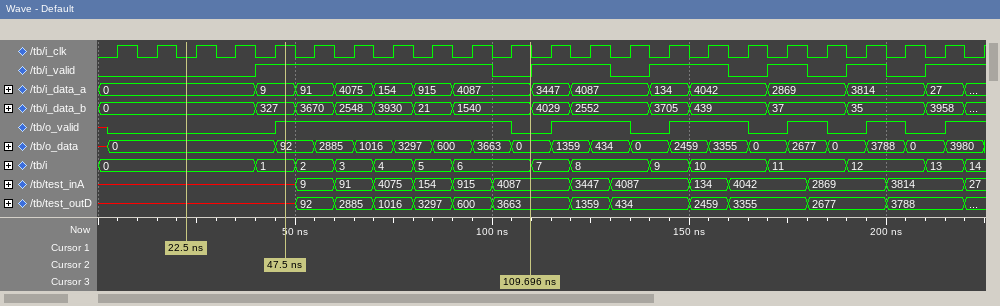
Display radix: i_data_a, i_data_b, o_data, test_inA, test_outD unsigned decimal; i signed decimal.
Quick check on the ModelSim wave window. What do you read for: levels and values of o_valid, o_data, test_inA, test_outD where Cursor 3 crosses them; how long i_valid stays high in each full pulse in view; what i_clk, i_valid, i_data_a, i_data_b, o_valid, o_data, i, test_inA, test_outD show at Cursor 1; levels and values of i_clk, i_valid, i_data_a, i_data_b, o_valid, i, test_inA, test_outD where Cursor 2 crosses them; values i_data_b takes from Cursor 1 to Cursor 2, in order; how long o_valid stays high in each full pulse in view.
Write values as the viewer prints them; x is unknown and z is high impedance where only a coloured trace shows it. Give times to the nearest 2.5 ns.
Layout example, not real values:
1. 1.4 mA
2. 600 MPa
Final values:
1. o_valid=0, o_data=0, test_inA=4087, test_outD=3663
2. 60 ns, 20 ns, 20 ns, 10 ns, 10 ns
3. i_clk=0, i_valid=0, i_data_a=0, i_data_b=0, o_valid=0, o_data=0, i=0, test_inA=x, test_outD=x
4. i_clk=1, i_valid=1, i_data_a=9, i_data_b=327, o_valid=1, i=1, test_inA=x, test_outD=x
5. 0, 327
6. 60 ns, 20 ns, 20 ns, 10 ns, 10 ns
